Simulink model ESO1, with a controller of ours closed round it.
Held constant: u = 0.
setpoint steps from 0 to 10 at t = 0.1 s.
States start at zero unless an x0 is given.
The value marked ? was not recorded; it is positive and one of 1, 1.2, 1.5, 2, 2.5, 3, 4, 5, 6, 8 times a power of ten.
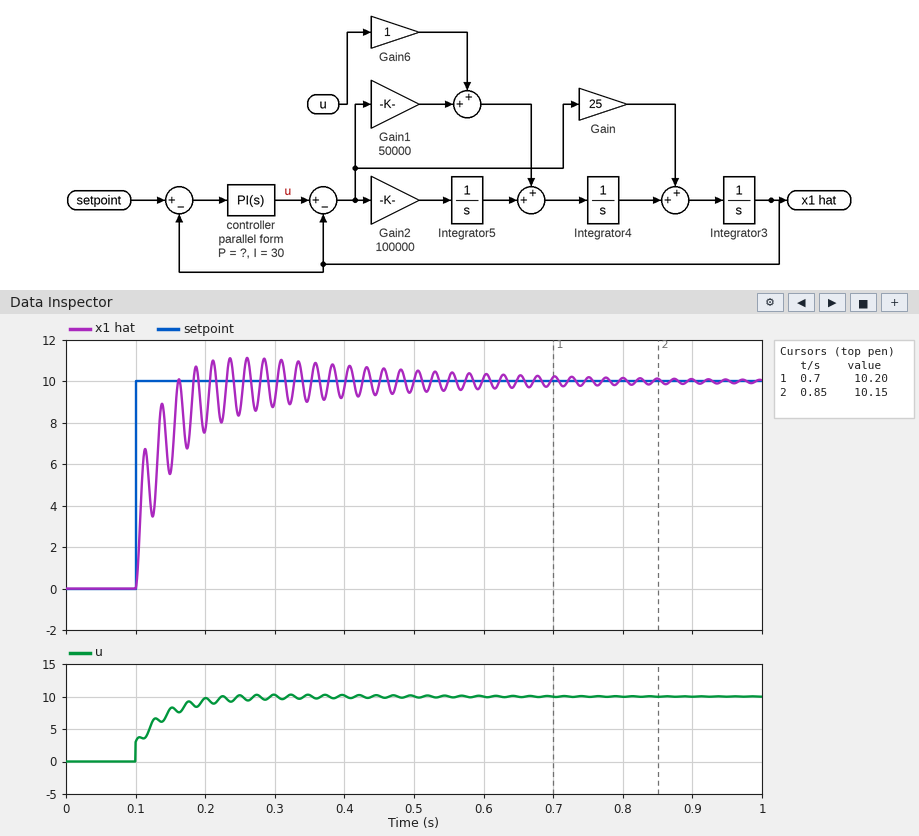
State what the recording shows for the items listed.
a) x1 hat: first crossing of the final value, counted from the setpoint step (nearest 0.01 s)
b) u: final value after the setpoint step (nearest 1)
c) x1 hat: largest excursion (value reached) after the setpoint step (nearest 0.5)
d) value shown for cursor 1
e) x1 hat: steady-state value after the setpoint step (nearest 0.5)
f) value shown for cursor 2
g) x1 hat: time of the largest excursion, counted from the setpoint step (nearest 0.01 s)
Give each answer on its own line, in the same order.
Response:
0.06 s
10
11.0
10.20
10.0
10.15
0.16 s
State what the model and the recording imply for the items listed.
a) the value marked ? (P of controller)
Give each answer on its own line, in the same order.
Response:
0.3
